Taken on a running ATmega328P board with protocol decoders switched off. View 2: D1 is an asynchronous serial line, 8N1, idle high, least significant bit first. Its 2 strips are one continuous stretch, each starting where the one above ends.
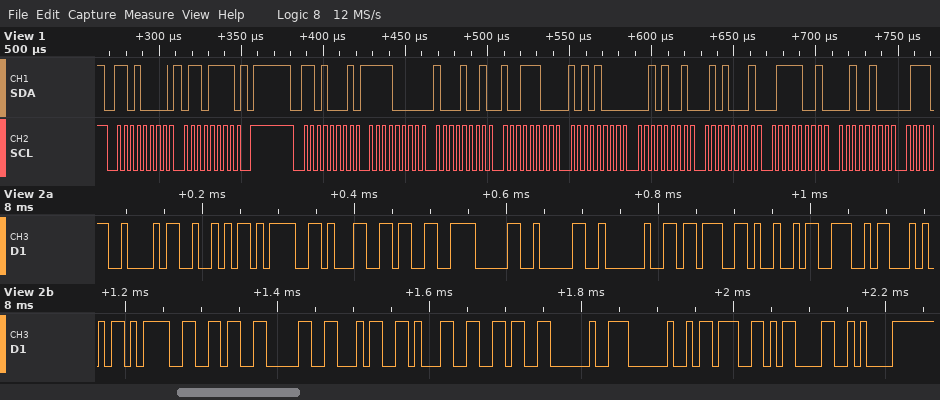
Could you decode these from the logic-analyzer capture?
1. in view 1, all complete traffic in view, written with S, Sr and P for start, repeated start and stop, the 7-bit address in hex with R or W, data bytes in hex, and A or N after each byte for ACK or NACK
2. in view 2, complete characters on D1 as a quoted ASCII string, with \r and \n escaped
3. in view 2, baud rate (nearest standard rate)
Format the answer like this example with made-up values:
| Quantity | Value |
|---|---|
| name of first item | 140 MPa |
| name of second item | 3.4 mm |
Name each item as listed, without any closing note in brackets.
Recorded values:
| Quantity | Value |
|---|---|
| in view 1, all complete traffic in view, written with S, Sr and P for start, repeated start and stop, the 7-bit address in hex with R or W, data bytes in hex, and A or N after each byte for ACK or NACK | S 68W A 6F A P S 68R A F0 A 89 A 9C A A8 A 29 A 51 A 79 A 24 A |
| in view 2, complete characters on D1 as a quoted ASCII string, with \r and \n escaped | "BR=1300 ;INT=60416  ;\r\n" |
| in view 2, baud rate | 115200 baud |
